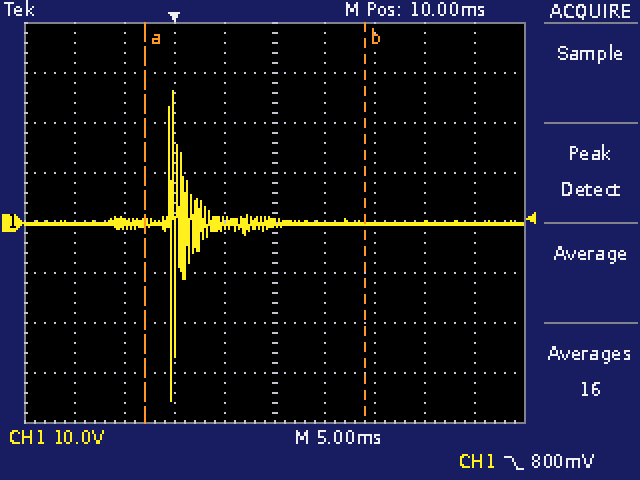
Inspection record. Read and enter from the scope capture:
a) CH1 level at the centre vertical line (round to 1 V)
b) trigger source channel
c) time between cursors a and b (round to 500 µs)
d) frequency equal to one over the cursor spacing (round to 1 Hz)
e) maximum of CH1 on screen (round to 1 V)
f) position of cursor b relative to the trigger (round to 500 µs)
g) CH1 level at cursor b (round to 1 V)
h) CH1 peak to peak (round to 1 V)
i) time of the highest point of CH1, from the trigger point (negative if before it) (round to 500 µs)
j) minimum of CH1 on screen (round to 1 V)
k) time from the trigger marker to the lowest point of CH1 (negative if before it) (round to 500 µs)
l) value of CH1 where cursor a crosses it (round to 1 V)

0 V
CH1
22.0 ms
45 Hz
26 V
+19.0 ms
0 V
62 V
0.0 ms
-36 V
-500 µs
0 V
